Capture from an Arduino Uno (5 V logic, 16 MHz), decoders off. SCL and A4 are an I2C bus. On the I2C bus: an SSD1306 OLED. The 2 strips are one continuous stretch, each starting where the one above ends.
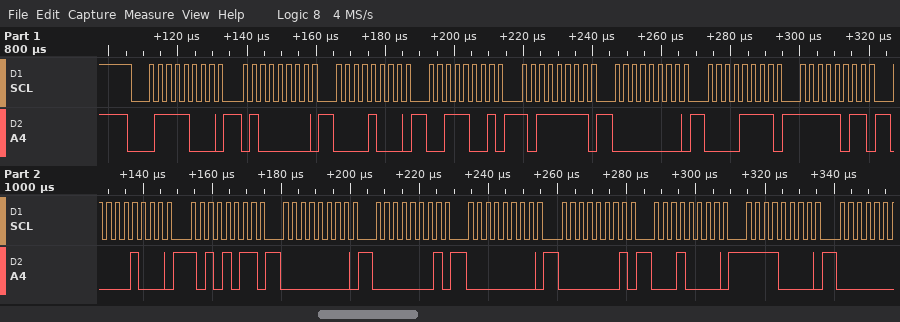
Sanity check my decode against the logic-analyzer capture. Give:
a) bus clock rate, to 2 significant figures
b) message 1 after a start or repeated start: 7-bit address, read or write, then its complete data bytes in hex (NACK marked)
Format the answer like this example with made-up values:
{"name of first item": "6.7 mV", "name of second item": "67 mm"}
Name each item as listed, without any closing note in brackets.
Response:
{"bus clock rate, to 2 significant figures": "400 kHz", "message 1 after a start or repeated start: 7-bit address, read or write, then its complete data bytes in hex": "0x3C write: 40 08 39 BF 00 0F FB 08 AB 00 01 00 01 10 F0"}
